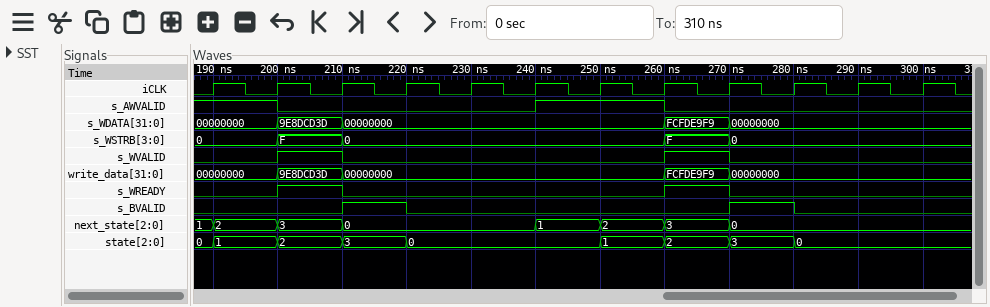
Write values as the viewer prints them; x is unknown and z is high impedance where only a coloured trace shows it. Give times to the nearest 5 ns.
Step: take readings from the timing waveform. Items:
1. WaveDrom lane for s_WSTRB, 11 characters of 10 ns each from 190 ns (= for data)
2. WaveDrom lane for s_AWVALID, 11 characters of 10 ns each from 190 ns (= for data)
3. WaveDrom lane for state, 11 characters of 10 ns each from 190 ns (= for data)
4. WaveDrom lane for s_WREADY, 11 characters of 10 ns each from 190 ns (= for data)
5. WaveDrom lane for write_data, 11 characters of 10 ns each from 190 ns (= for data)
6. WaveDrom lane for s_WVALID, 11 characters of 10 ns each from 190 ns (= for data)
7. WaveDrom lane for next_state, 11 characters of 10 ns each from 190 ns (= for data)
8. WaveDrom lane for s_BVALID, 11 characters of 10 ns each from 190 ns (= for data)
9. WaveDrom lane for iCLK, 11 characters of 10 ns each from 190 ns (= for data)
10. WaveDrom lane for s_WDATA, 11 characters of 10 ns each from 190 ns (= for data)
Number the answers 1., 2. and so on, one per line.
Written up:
1. {name: 's_WSTRB', wave: '===....==..', data: '0 F 0 F 0'}
2. {name: 's_AWVALID', wave: '10...1.0...'}
3. {name: 'state', wave: '====..====.', data: '1 2 3 0 1 2 3 0'}
4. {name: 's_WREADY', wave: '010....10..'}
5. {name: 'write_data', wave: '===....==..', data: '00000000 9E8DCD3D 00000000 FCFDE9F9 00000000'}
6. {name: 's_WVALID', wave: '010....10..'}
7. {name: 'next_state', wave: '===..====..', data: '2 3 0 1 2 3 0'}
8. {name: 's_BVALID', wave: '0.10....10.'}
9. {name: 'iCLK', wave: 'p..........'}
10. {name: 's_WDATA', wave: '===....==..', data: '00000000 9E8DCD3D 00000000 FCFDE9F9 00000000'}
